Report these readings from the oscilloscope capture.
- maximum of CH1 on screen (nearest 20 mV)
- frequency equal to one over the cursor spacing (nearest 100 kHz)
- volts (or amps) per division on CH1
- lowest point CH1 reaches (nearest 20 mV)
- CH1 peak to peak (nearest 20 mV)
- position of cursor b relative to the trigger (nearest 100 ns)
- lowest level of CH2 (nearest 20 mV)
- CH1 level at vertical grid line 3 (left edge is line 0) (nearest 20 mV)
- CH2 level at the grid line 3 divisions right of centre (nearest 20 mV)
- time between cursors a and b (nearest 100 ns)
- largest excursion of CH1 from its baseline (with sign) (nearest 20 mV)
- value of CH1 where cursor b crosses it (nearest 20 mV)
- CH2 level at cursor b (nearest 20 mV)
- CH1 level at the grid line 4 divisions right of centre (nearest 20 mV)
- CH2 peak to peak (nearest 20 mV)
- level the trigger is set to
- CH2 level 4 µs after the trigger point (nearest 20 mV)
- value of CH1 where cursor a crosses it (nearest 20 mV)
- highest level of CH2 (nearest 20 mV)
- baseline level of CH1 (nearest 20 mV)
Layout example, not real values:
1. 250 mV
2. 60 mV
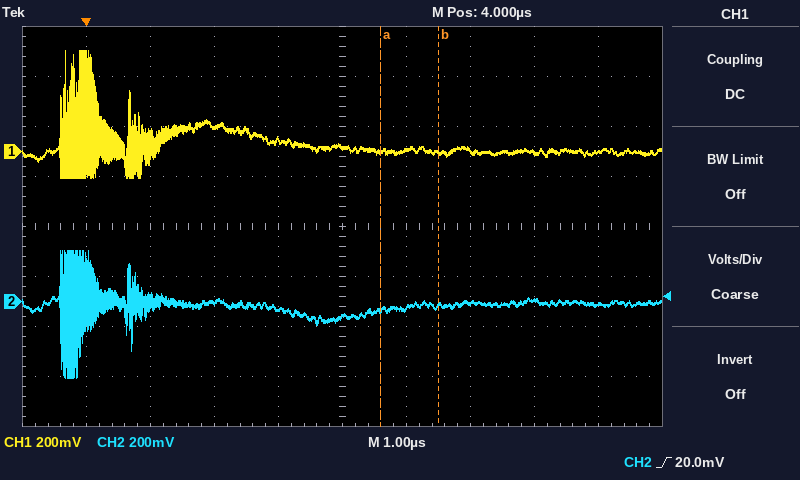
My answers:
1. 400 mV
2. 1.1 MHz
3. 200 mV
4. -100 mV
5. 500 mV
6. +5.5 µs
7. -300 mV
8. 100 mV
9. 0 mV
10. 900 ns
11. +400 mV
12. 0 mV
13. -20 mV
14. 0 mV
15. 500 mV
16. 20.0 mV
17. -60 mV
18. 0 mV
19. 200 mV
20. 0 mV
